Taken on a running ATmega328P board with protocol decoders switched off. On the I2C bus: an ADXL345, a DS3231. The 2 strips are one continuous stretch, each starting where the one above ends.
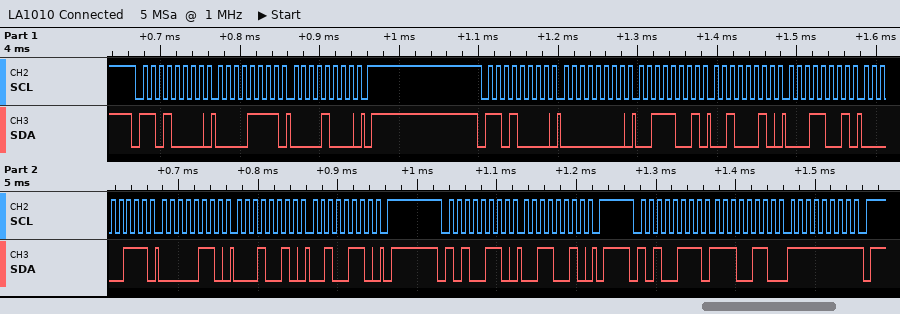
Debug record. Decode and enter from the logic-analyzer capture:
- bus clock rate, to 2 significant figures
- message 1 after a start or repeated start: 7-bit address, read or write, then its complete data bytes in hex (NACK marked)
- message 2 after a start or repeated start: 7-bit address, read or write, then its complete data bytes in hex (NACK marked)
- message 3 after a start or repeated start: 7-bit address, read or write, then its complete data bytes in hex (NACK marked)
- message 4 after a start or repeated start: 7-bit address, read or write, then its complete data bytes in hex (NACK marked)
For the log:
100 kHz
0x68 write: 0F 08
0x68 write: 00 39 22 19 07 06 12 26
0x53 write: 32
0x53 read: E6 FF NACK
